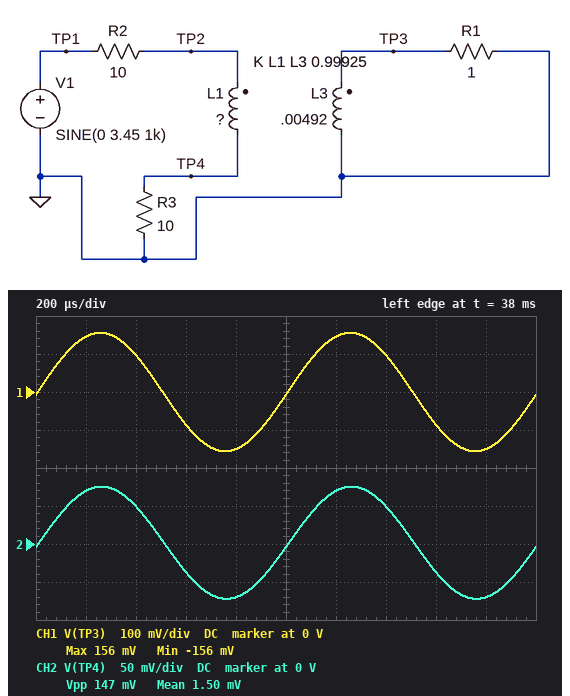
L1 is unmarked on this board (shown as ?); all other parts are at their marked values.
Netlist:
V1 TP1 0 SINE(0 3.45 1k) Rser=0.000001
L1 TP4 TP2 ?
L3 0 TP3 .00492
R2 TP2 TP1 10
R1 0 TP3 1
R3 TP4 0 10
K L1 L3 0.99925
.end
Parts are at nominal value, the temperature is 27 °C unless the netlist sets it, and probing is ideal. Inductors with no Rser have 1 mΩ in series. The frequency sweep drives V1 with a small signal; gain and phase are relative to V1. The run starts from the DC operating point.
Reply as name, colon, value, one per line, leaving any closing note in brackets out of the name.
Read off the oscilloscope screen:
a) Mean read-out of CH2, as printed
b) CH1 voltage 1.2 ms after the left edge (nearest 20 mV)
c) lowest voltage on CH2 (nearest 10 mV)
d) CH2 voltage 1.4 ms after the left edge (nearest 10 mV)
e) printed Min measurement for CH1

Mean read-out of CH2, as printed: 1.50 mV
CH1 voltage 1.2 ms after the left edge: 140 mV
lowest voltage on CH2: -70 mV
CH2 voltage 1.4 ms after the left edge: 50 mV
printed Min measurement for CH1: -156 mV
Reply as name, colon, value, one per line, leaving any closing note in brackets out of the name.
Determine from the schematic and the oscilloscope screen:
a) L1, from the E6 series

L1, from the E6 series: 2.2 H
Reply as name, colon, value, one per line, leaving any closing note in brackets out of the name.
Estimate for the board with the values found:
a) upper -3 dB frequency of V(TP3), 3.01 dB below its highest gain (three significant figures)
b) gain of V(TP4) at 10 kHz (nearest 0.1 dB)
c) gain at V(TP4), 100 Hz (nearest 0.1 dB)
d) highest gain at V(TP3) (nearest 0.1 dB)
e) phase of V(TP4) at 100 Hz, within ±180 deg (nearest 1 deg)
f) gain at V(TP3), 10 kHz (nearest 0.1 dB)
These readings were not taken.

upper -3 dB frequency of V(TP3), 3.01 dB below its highest gain: 22.6 kHz
gain of V(TP4) at 10 kHz: -34.2 dB
gain at V(TP4), 100 Hz: -33.0 dB
highest gain at V(TP3): -26.9 dB
phase of V(TP4) at 100 Hz, within ±180 deg: -17 deg
gain at V(TP3), 10 kHz: -27.7 dB
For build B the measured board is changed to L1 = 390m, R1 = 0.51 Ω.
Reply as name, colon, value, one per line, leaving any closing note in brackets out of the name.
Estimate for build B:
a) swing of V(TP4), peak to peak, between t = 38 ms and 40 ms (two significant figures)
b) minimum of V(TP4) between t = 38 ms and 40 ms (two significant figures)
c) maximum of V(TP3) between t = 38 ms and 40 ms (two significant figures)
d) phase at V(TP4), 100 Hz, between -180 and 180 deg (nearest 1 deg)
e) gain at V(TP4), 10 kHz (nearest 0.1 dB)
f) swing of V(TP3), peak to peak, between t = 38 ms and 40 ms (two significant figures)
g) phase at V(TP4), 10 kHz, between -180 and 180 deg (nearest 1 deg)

swing of V(TP4), peak to peak, between t = 38 ms and 40 ms: 1.1 V
minimum of V(TP4) between t = 38 ms and 40 ms: -570 mV
maximum of V(TP3) between t = 38 ms and 40 ms: 260 mV
phase at V(TP4), 100 Hz, between -180 and 180 deg: -7 deg
gain at V(TP4), 10 kHz: -17.0 dB
swing of V(TP3), peak to peak, between t = 38 ms and 40 ms: 520 mV
phase at V(TP4), 10 kHz, between -180 and 180 deg: -31 deg
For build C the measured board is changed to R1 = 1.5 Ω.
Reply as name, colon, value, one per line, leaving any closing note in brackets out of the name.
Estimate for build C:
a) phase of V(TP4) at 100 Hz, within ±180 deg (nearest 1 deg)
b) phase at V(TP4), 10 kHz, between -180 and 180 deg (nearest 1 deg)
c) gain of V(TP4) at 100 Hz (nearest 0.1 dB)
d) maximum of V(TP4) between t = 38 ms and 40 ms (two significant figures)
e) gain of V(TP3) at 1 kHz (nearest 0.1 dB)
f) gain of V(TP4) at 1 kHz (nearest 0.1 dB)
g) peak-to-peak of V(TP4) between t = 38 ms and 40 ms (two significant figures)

phase of V(TP4) at 100 Hz, within ±180 deg: -25 deg
phase at V(TP4), 10 kHz, between -180 and 180 deg: -17 deg
gain of V(TP4) at 100 Hz: -35.9 dB
maximum of V(TP4) between t = 38 ms and 40 ms: 52 mV
gain of V(TP3) at 1 kHz: -26.8 dB
gain of V(TP4) at 1 kHz: -36.8 dB
peak-to-peak of V(TP4) between t = 38 ms and 40 ms: 100 mV
